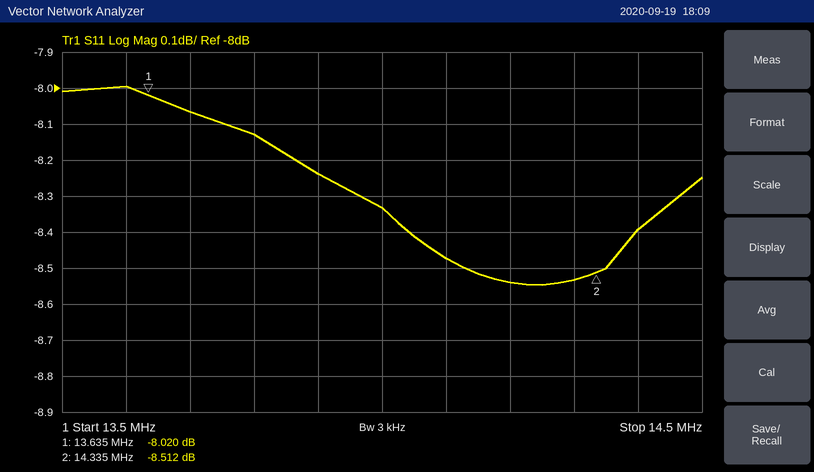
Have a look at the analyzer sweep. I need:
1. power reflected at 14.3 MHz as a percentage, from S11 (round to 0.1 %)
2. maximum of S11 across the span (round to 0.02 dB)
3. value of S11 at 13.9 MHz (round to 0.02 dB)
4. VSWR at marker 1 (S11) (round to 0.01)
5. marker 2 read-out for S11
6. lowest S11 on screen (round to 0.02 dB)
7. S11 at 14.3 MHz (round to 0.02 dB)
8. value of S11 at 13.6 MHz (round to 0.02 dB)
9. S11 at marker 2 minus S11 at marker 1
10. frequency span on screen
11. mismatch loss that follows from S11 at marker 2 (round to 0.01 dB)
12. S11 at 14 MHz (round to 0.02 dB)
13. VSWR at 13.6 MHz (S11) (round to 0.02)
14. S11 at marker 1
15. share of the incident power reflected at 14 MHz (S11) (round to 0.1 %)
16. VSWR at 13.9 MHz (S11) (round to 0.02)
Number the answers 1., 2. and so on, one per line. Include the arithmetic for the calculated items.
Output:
1. 10^(-8.54/10) ≈ 14.0 %
2. -8.00 dB
3. -8.24 dB
4. (1 + 0.3972)/(1 − 0.3972) ≈ 2.32
5. -8.512 dB
6. -8.54 dB
7. -8.54 dB
8. -8.00 dB
9. -8.512 − (-8.02) = -0.492 dB
10. 1 MHz
11. −10 log10(1 − 10^(-8.512/10)) ≈ 0.66 dB
12. -8.34 dB
13. |Γ| = 10^(-8/20) = 0.3981; VSWR = (1 + 0.3981)/(1 − 0.3981) ≈ 2.32
14. -8.020 dB
15. 10^(-8.34/10) ≈ 14.7 %
16. |Γ| = 10^(-8.24/20) = 0.3873; VSWR = (1 + 0.3873)/(1 − 0.3873) ≈ 2.26
